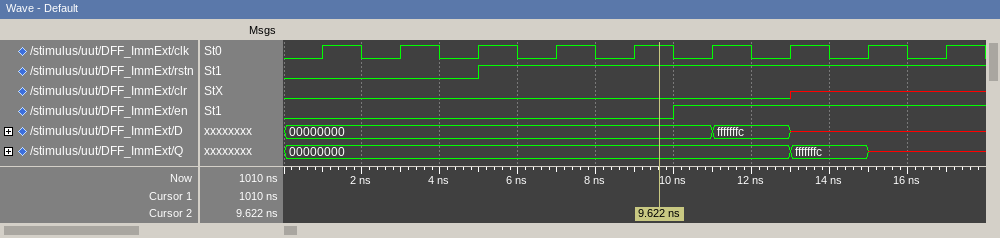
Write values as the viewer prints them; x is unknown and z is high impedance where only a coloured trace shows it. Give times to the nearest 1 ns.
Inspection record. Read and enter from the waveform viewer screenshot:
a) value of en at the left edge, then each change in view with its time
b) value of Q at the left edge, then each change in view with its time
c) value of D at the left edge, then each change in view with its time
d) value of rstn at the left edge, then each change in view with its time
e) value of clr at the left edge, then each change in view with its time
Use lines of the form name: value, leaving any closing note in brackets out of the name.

value of en at the left edge, then each change in view with its time: 0, 1 at 10 ns
value of Q at the left edge, then each change in view with its time: 00000000, fffffffc at 13 ns, x at 15 ns
value of D at the left edge, then each change in view with its time: 00000000, fffffffc at 11 ns, x at 13 ns
value of rstn at the left edge, then each change in view with its time: 0, 1 at 5 ns
value of clr at the left edge, then each change in view with its time: 0, x at 13 ns
